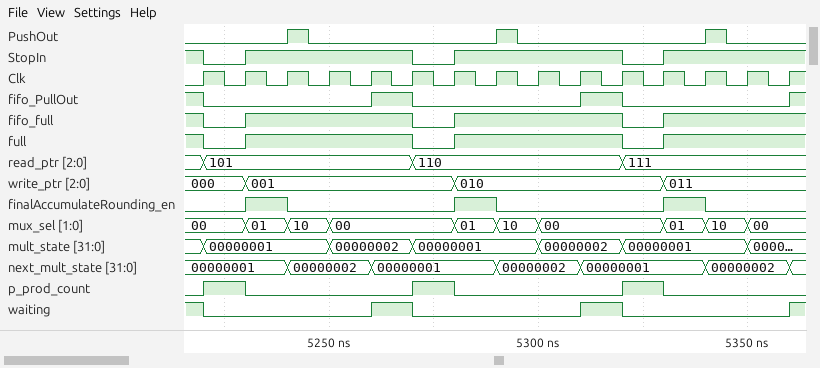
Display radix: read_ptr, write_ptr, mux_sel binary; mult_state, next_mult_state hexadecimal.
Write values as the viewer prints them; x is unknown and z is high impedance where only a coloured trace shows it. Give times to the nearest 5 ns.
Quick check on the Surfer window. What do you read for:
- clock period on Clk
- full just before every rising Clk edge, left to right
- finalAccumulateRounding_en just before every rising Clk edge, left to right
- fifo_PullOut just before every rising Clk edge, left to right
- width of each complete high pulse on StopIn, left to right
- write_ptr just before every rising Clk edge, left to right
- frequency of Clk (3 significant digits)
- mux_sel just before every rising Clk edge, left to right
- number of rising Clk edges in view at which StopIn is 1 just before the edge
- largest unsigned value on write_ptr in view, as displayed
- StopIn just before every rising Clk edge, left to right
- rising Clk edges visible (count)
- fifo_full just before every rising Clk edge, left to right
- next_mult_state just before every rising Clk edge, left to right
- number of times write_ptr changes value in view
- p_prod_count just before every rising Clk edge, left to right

10 ns
1 0 1 1 1 1 0 1 1 1 1 0 1 1 1
0 0 1 0 0 0 0 1 0 0 0 0 1 0 0
1 0 0 0 0 1 0 0 0 0 1 0 0 0 0
40 ns, 40 ns
000, 000, 001, 001, 001, 001, 001, 010, 010, 010, 010, 010, 011, 011, 011
100 MHz
00, 00, 01, 10, 00, 00, 00, 01, 10, 00, 00, 00, 01, 10, 00
12
011
1 0 1 1 1 1 0 1 1 1 1 0 1 1 1
15
1 0 1 1 1 1 0 1 1 1 1 0 1 1 1
00000001, 00000001, 00000001, 00000002, 00000002, 00000001, 00000001, 00000001, 00000002, 00000002, 00000001, 00000001, 00000001, 00000002, 00000002
3
0 1 0 0 0 0 1 0 0 0 0 1 0 0 0
